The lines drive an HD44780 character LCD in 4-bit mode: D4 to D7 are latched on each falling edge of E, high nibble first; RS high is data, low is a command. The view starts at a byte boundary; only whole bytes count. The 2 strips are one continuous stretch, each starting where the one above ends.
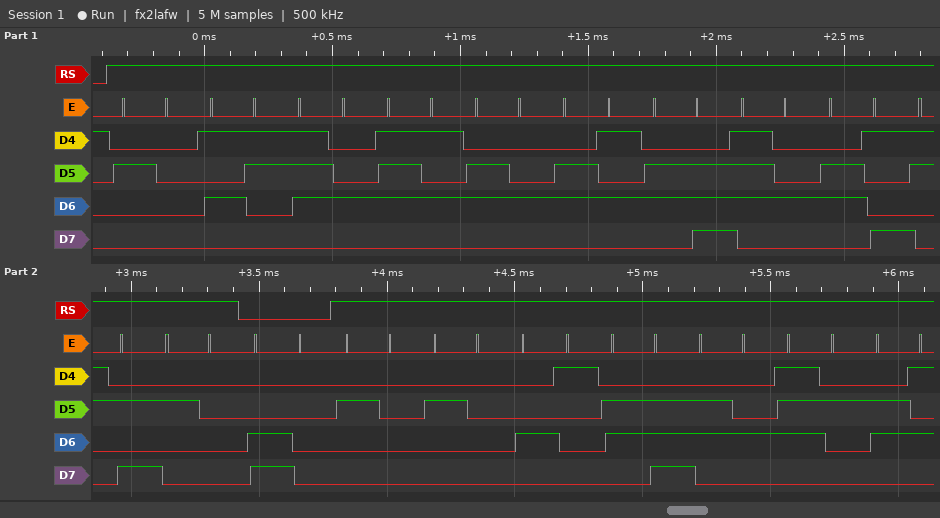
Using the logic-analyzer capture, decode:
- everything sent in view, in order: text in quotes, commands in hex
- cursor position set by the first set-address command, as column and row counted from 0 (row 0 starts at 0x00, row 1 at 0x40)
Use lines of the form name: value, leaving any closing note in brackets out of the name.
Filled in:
everything sent in view, in order: text in quotes, commands in hex: " Studenti: " 0xC0 "  Andre"
cursor position set by the first set-address command, as column and row counted from 0: column 0, row 1
